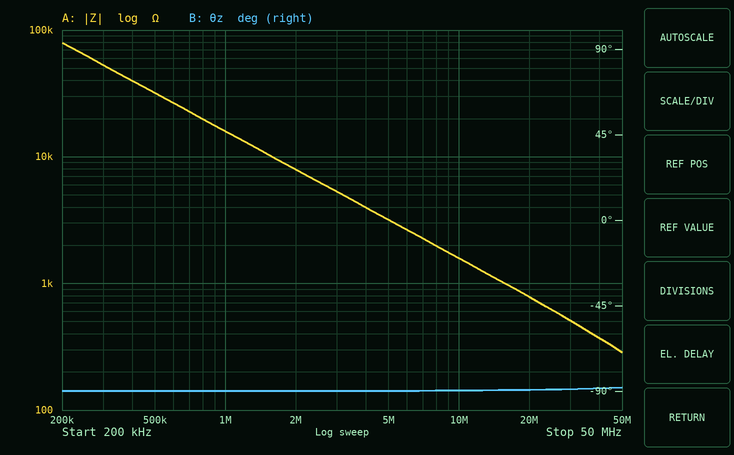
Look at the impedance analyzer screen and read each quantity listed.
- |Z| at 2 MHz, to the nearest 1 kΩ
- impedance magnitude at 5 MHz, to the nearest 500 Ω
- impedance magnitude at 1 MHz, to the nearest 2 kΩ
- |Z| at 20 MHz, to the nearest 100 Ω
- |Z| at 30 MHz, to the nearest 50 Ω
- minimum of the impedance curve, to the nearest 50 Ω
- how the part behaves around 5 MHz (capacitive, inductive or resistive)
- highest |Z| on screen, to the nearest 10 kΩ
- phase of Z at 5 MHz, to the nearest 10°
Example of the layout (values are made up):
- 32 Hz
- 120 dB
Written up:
- 8 kΩ
- 3.0 kΩ
- 16 kΩ
- 800 Ω
- 500 Ω
- 300 Ω
- capacitive
- 80 kΩ
- -90°
